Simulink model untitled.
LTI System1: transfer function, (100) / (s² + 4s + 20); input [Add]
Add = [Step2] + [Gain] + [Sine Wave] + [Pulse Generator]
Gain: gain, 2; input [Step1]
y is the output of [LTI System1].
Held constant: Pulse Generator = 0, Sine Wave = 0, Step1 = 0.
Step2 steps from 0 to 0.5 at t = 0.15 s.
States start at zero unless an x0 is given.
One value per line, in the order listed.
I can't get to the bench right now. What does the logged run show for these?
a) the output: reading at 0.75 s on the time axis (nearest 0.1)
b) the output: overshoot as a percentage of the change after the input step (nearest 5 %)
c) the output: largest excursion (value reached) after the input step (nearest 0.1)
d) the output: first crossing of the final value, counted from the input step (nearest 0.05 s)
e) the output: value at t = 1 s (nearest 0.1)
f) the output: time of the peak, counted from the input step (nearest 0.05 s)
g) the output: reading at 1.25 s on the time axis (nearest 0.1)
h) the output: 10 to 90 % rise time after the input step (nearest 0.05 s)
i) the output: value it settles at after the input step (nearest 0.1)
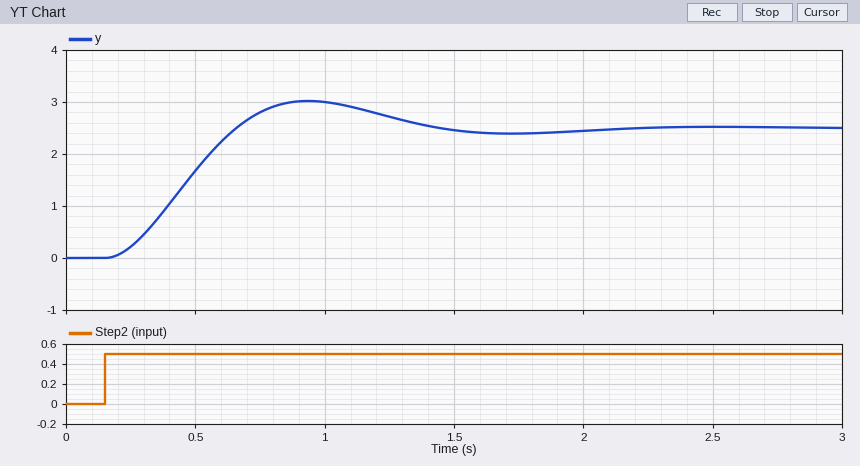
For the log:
2.8
20 %
3.0
0.50 s
3.0
0.80 s
2.7
0.35 s
2.5
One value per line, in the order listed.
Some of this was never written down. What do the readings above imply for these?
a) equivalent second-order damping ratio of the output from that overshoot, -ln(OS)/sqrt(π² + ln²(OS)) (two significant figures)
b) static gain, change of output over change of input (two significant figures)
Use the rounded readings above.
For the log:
0.46
5.0
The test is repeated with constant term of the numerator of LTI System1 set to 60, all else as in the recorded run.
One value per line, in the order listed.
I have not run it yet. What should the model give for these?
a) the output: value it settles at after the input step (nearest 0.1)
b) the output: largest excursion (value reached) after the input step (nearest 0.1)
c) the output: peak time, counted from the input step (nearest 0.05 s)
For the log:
1.5
1.8
0.80 s
